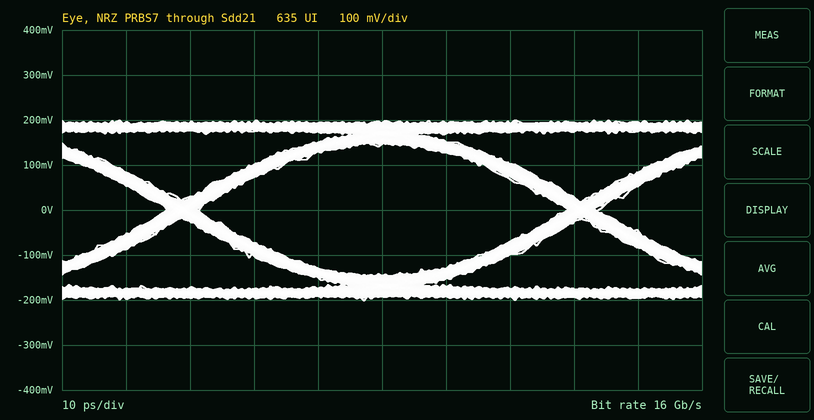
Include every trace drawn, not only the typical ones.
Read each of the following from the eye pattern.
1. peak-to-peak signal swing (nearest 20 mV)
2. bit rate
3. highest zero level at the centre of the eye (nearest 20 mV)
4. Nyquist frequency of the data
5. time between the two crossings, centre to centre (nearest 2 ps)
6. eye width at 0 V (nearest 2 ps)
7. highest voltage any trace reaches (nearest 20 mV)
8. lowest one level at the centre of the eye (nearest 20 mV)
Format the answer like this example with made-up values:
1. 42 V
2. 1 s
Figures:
1. 400 mV
2. 16 Gb/s
3. -140 mV
4. 8 GHz
5. 62 ps
6. 58 ps
7. 200 mV
8. 140 mV
